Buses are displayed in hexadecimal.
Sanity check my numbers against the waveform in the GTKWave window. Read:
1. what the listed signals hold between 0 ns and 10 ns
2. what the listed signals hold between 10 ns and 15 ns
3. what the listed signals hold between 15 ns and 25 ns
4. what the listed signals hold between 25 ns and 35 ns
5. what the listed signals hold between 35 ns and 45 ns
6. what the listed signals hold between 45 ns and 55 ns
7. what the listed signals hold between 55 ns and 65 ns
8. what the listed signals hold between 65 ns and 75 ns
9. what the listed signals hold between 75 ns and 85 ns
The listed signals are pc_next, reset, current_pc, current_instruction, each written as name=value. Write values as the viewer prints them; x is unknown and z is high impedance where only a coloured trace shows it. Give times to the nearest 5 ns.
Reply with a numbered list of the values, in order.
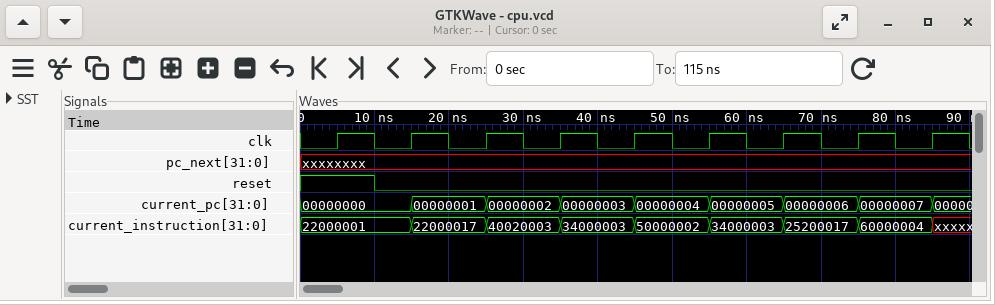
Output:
1. pc_next=xxxxxxxx, reset=1, current_pc=00000000, current_instruction=22000001
2. pc_next=xxxxxxxx, reset=0, current_pc=00000000, current_instruction=22000001
3. pc_next=xxxxxxxx, reset=0, current_pc=00000001, current_instruction=22000017
4. pc_next=xxxxxxxx, reset=0, current_pc=00000002, current_instruction=40020003
5. pc_next=xxxxxxxx, reset=0, current_pc=00000003, current_instruction=34000003
6. pc_next=xxxxxxxx, reset=0, current_pc=00000004, current_instruction=50000002
7. pc_next=xxxxxxxx, reset=0, current_pc=00000005, current_instruction=34000003
8. pc_next=xxxxxxxx, reset=0, current_pc=00000006, current_instruction=25200017
9. pc_next=xxxxxxxx, reset=0, current_pc=00000007, current_instruction=60000004
